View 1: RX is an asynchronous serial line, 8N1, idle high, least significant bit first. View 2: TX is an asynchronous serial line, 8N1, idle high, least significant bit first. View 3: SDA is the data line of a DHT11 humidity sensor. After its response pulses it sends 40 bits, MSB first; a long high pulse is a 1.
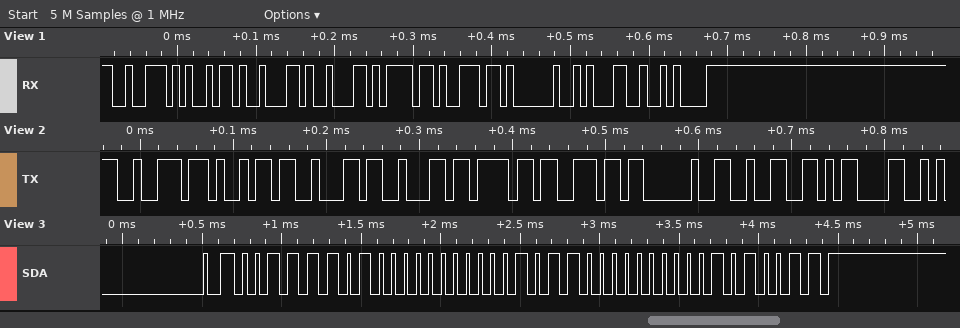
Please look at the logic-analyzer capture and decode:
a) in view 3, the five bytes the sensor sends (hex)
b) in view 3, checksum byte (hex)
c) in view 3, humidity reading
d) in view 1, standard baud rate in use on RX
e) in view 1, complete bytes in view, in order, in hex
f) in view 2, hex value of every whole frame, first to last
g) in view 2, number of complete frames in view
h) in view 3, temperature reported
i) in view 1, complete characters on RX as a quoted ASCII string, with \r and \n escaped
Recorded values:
3D 00 16 00 53
0x53
61 %
115200 baud
72 69 62 62 6F 6E 20 31 0A
0x72 0x69 0x62 0x62 0x6F 0x6E 0x20 0x32 0x0D
9
22.0 °C
"ribbon 1\n"
